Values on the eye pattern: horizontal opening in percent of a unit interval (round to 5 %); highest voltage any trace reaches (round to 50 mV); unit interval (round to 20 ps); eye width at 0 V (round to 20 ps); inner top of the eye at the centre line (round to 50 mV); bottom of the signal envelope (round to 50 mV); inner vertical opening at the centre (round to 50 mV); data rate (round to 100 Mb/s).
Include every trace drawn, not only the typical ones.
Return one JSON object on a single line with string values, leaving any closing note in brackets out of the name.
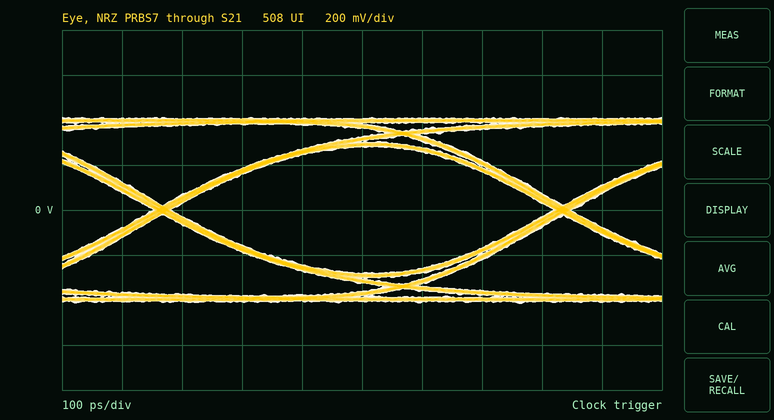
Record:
{"horizontal opening in percent of a unit interval": "95 %", "highest voltage any trace reaches": "400 mV", "unit interval": "660 ps", "eye width at 0 V": "640 ps", "inner top of the eye at the centre line": "300 mV", "bottom of the signal envelope": "-400 mV", "inner vertical opening at the centre": "550 mV", "data rate": "1.5 Gb/s"}
